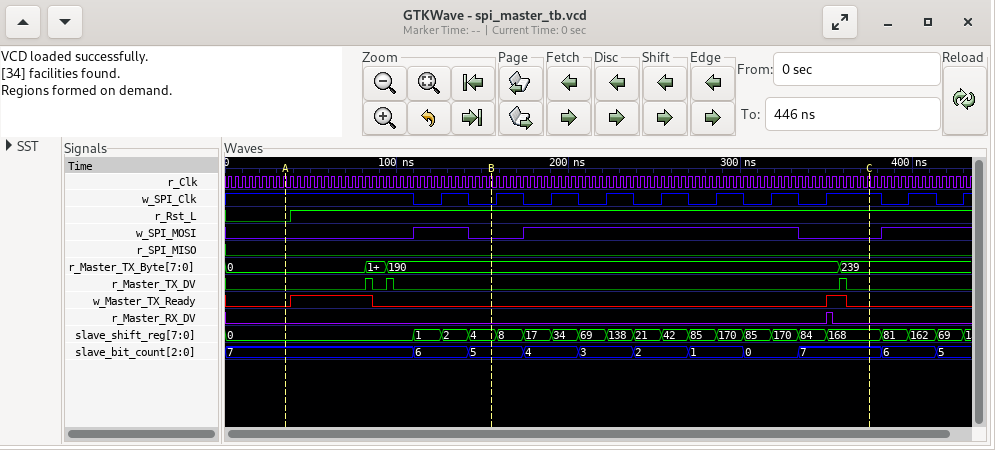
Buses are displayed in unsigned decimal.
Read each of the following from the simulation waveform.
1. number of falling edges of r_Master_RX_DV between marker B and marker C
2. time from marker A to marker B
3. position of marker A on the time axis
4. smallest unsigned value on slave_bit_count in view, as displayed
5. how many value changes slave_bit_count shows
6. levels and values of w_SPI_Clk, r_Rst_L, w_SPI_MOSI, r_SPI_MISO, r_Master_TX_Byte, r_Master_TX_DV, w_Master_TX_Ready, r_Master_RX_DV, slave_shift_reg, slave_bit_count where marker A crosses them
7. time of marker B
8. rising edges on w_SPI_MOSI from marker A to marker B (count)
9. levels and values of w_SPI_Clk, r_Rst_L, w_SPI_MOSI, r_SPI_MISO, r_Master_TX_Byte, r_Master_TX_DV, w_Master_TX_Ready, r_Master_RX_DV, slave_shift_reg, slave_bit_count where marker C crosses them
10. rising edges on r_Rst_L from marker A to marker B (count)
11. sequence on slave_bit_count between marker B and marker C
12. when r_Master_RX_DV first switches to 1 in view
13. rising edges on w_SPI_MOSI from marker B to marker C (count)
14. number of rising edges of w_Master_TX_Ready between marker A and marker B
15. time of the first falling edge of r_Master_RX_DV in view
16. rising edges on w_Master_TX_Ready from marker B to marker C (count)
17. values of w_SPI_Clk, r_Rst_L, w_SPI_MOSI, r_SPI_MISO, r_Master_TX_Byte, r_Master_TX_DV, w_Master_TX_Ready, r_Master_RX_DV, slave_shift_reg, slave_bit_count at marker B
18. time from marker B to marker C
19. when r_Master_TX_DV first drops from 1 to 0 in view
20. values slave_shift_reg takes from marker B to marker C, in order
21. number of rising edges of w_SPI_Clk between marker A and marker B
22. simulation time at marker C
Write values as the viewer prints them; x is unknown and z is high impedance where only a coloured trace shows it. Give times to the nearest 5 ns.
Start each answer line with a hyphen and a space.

- 1
- 120 ns
- 35 ns
- 0
- 10
- w_SPI_Clk=1, r_Rst_L=0, w_SPI_MOSI=0, r_SPI_MISO=0, r_Master_TX_Byte=0, r_Master_TX_DV=0, w_Master_TX_Ready=0, r_Master_RX_DV=0, slave_shift_reg=0, slave_bit_count=7
- 155 ns
- 1
- w_SPI_Clk=1, r_Rst_L=1, w_SPI_MOSI=0, r_SPI_MISO=0, r_Master_TX_Byte=239, r_Master_TX_DV=0, w_Master_TX_Ready=0, r_Master_RX_DV=0, slave_shift_reg=168, slave_bit_count=7
- 1
- 5, 4, 3, 2, 1, 0, 7
- 350 ns
- 1
- 1
- 355 ns
- 1
- w_SPI_Clk=0, r_Rst_L=1, w_SPI_MOSI=0, r_SPI_MISO=0, r_Master_TX_Byte=190, r_Master_TX_DV=0, w_Master_TX_Ready=0, r_Master_RX_DV=0, slave_shift_reg=4, slave_bit_count=5
- 220 ns
- 85 ns
- 4, 8, 17, 34, 69, 138, 21, 42, 85, 170, 85, 170, 84, 168
- 1
- 375 ns
